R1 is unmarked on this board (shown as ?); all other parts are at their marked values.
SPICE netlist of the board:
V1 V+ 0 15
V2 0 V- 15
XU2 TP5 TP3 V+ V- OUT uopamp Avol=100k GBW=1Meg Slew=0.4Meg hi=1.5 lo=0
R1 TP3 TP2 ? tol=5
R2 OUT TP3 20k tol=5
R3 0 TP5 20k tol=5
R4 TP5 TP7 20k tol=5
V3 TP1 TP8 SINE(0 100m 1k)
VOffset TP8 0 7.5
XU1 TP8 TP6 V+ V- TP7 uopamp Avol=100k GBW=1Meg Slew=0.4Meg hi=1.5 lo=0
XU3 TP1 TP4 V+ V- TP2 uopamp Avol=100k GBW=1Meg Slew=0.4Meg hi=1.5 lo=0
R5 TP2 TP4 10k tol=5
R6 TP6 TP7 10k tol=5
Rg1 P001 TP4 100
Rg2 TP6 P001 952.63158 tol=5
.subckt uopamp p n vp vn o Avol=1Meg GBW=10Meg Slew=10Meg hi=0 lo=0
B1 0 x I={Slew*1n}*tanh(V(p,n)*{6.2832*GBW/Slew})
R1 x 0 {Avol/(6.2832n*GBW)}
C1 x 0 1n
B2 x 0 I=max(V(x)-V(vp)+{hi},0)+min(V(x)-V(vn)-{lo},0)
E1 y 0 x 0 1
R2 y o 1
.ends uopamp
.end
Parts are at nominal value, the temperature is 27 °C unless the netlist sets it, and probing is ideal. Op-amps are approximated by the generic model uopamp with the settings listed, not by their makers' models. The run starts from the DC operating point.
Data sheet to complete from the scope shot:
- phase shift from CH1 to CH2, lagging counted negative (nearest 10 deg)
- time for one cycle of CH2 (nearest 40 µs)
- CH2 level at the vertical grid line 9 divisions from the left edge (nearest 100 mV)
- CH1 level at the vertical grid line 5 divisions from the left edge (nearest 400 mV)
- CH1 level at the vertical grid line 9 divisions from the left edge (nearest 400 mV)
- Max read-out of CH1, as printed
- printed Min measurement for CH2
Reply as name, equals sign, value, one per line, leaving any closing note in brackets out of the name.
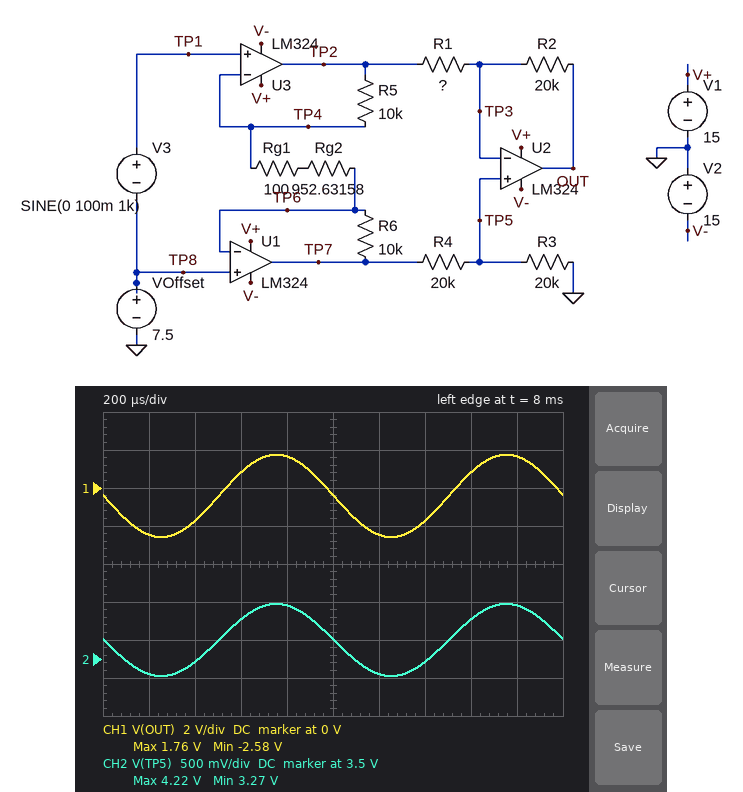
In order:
phase shift from CH1 to CH2, lagging counted negative = 0 deg
time for one cycle of CH2 = 1.00 ms
CH2 level at the vertical grid line 9 divisions from the left edge = 4.2 V
CH1 level at the vertical grid line 5 divisions from the left edge = -400 mV
CH1 level at the vertical grid line 9 divisions from the left edge = 1.6 V
Max read-out of CH1, as printed = 1.76 V
printed Min measurement for CH2 = 3.27 V
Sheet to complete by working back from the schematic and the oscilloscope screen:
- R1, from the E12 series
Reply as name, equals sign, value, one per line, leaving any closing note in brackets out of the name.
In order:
R1, from the E12 series = 18 kΩ
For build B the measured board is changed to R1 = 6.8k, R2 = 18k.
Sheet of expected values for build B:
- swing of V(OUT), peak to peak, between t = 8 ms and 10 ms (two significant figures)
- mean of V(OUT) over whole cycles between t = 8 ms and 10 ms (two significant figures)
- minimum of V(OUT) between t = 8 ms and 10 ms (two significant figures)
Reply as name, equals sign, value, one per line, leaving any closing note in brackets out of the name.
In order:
swing of V(OUT), peak to peak, between t = 8 ms and 10 ms = 9.0 V
mean of V(OUT) over whole cycles between t = 8 ms and 10 ms = -6.2 V
minimum of V(OUT) between t = 8 ms and 10 ms = -11 V
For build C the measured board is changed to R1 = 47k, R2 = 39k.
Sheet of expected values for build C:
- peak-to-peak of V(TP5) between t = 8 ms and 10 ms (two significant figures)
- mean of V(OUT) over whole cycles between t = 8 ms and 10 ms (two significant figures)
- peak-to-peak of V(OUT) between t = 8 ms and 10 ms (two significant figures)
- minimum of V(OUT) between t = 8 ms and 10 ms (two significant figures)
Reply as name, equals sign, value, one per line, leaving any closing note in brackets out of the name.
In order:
peak-to-peak of V(TP5) between t = 8 ms and 10 ms = 950 mV
mean of V(OUT) over whole cycles between t = 8 ms and 10 ms = 640 mV
peak-to-peak of V(OUT) between t = 8 ms and 10 ms = 3.5 V
minimum of V(OUT) between t = 8 ms and 10 ms = -1.1 V
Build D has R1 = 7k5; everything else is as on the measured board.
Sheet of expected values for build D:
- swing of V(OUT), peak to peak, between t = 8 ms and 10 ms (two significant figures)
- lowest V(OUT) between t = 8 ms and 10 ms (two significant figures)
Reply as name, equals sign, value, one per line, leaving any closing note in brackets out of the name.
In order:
swing of V(OUT), peak to peak, between t = 8 ms and 10 ms = 9.1 V
lowest V(OUT) between t = 8 ms and 10 ms = -11 V
